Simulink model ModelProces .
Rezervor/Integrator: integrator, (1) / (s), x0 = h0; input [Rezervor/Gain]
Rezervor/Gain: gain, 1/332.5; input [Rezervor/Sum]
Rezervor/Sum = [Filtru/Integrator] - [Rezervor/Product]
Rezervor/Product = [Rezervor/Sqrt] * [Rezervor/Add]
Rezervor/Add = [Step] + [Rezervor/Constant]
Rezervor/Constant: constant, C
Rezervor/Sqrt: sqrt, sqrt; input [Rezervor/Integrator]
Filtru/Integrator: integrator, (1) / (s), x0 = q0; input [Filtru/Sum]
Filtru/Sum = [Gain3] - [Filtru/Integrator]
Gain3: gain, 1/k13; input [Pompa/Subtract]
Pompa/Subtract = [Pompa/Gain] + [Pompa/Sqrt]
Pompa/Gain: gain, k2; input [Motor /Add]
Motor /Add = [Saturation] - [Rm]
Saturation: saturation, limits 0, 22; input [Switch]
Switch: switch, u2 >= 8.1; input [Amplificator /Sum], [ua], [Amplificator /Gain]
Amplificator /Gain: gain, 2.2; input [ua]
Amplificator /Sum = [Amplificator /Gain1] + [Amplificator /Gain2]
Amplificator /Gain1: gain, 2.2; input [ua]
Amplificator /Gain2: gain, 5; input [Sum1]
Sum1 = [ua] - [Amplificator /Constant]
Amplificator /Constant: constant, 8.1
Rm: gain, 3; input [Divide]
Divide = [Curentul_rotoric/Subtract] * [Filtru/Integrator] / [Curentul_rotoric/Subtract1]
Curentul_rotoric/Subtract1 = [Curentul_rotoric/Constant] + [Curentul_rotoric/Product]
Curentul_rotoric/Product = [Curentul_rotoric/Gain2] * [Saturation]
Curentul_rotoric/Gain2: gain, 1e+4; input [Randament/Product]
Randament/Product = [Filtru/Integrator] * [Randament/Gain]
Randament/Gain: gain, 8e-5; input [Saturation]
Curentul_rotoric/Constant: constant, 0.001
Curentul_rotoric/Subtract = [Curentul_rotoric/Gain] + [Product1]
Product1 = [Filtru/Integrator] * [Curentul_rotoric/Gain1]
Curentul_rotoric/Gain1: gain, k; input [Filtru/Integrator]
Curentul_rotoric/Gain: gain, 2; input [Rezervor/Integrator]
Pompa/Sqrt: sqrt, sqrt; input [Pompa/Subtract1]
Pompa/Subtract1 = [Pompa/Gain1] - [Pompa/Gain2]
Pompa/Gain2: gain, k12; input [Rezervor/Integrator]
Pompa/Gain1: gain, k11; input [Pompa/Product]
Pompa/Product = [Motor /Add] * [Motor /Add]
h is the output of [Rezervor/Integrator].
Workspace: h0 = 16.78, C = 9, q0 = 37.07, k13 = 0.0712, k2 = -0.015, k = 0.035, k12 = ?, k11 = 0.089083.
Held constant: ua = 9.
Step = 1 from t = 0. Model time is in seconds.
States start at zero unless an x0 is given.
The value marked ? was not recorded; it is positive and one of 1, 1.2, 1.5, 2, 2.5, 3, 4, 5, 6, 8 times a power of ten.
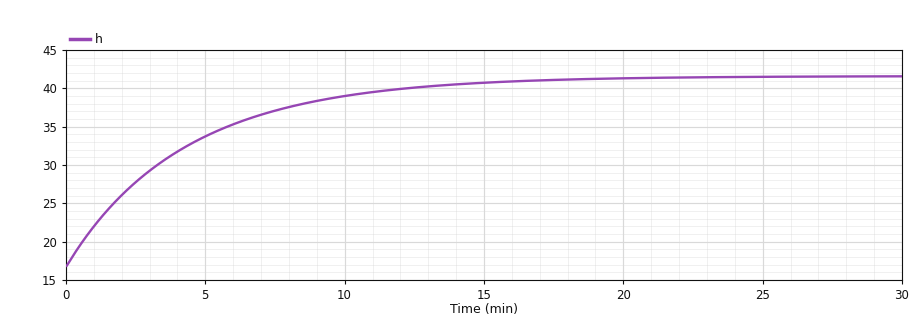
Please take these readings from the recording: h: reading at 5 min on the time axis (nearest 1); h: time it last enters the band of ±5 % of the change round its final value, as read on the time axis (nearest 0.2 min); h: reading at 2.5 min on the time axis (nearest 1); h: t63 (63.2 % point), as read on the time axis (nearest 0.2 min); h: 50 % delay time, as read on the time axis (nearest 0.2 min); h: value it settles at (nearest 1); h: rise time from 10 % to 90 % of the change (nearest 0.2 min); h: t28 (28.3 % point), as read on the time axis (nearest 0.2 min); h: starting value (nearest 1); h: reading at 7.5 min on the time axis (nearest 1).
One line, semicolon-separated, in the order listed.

34; 13.4 min; 28; 4.4 min; 3.0 min; 42; 9.8 min; 1.4 min; 17; 37
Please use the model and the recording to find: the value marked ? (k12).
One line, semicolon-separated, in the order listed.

0.3
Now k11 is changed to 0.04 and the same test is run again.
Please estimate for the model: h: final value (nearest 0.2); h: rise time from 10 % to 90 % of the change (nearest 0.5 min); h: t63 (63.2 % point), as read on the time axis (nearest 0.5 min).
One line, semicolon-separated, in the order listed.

19.6; 7.0 min; 3.0 min
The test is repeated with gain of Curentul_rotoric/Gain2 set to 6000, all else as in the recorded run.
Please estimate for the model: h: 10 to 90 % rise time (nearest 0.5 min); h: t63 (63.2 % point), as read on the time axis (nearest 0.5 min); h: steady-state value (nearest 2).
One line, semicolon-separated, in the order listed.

9.5 min; 4.0 min; 38
